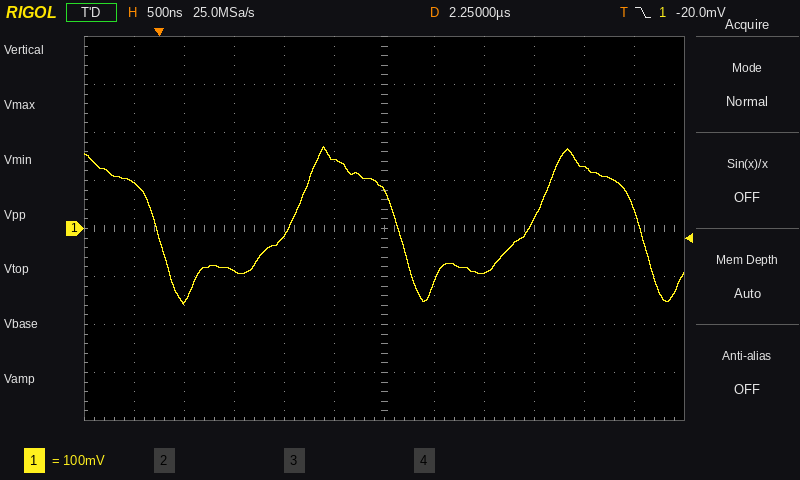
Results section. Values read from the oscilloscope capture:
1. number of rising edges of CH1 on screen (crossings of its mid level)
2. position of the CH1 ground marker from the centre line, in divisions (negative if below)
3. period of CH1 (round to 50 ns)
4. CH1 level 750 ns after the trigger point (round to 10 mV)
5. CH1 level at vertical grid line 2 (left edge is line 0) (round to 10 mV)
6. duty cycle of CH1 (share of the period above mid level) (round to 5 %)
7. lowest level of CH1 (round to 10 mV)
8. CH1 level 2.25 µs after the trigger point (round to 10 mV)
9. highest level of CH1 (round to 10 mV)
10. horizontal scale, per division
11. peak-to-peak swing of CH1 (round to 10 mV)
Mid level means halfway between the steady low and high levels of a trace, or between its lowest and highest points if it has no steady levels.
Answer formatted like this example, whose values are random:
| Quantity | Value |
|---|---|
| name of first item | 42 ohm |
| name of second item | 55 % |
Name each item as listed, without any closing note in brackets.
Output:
| Quantity | Value |
|---|---|
| number of rising edges of CH1 on screen | 2 |
| position of the CH1 ground marker from the centre line, in divisions | 0.0 div |
| period of CH1 | 2.40 µs |
| CH1 level 750 ns after the trigger point | -90 mV |
| CH1 level at vertical grid line 2 (left edge is line 0) | -150 mV |
| duty cycle of CH1 (share of the period above mid level) | 45 % |
| lowest level of CH1 | -160 mV |
| CH1 level 2.25 µs after the trigger point | 80 mV |
| highest level of CH1 | 170 mV |
| horizontal scale, per division | 500 ns |
| peak-to-peak swing of CH1 | 330 mV |
